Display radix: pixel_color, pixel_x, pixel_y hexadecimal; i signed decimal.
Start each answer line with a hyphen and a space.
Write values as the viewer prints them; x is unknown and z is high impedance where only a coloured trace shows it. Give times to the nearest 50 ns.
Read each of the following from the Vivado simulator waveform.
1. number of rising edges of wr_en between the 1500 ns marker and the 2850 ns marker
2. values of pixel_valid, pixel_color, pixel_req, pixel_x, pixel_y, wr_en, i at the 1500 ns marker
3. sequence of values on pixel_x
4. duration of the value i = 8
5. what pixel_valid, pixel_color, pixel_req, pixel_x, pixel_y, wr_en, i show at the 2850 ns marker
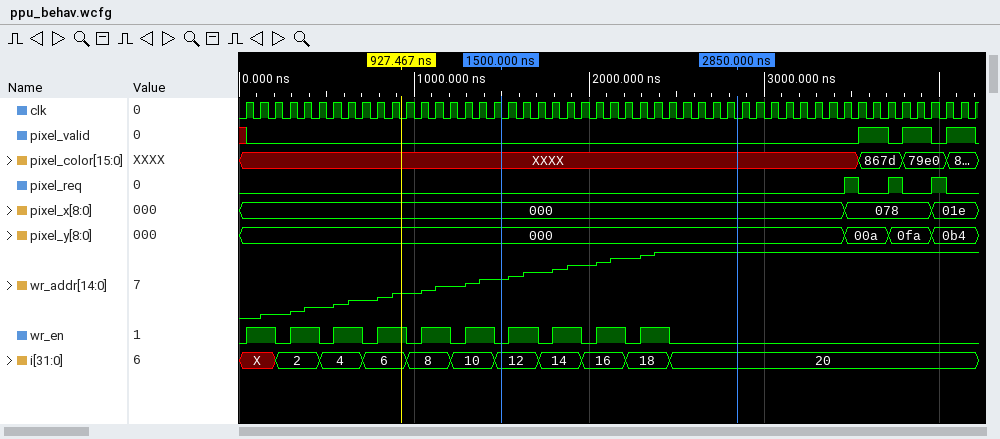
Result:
- 4
- pixel_valid=0, pixel_color=XXXX, pixel_req=0, pixel_x=000, pixel_y=000, wr_en=0, i=12
- 000, 078, 01e
- 250 ns
- pixel_valid=0, pixel_color=XXXX, pixel_req=0, pixel_x=000, pixel_y=000, wr_en=0, i=20
